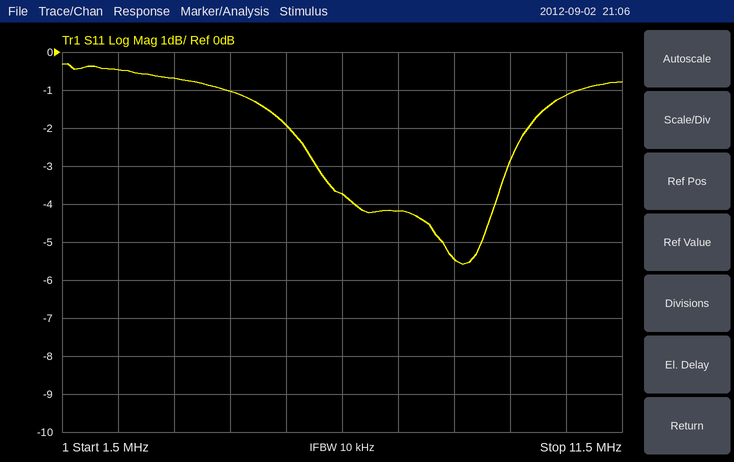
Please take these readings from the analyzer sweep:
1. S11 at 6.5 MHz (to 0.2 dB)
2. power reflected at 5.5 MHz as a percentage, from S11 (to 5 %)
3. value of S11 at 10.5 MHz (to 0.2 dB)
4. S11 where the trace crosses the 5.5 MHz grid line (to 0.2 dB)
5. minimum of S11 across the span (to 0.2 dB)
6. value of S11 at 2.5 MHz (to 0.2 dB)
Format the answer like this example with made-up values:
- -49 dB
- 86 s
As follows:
- -3.8 dB
- 65 %
- -1.2 dB
- -2.0 dB
- -5.6 dB
- -0.4 dB
